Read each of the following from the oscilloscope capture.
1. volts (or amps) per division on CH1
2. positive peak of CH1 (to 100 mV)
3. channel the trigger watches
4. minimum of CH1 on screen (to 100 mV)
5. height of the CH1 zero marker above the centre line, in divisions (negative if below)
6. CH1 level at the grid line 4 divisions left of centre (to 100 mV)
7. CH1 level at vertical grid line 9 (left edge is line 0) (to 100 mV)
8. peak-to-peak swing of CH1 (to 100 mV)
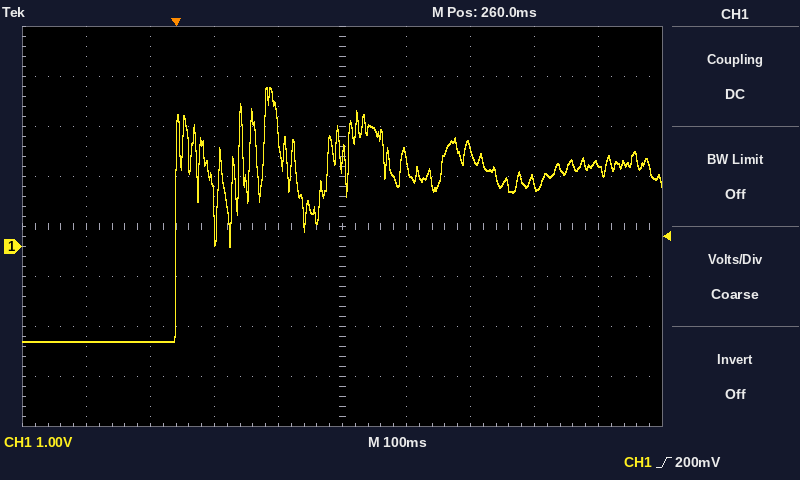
1 V
3.2 V
CH1
-1.9 V
-0.4 div
-1.9 V
1.7 V
5.1 V
